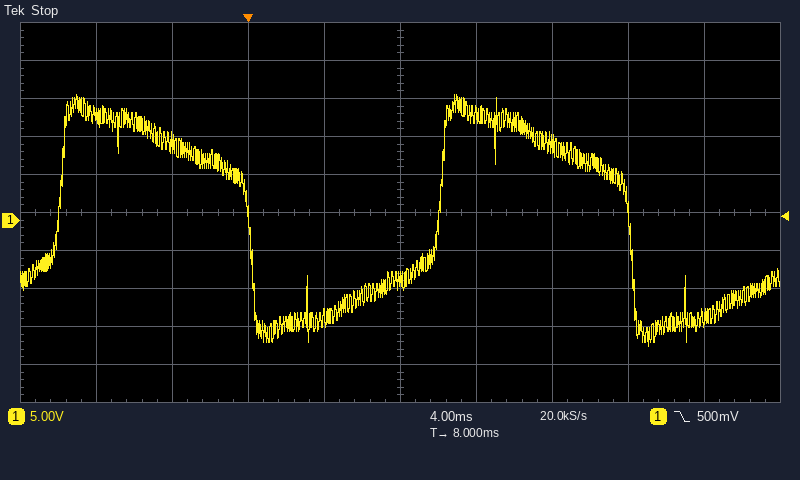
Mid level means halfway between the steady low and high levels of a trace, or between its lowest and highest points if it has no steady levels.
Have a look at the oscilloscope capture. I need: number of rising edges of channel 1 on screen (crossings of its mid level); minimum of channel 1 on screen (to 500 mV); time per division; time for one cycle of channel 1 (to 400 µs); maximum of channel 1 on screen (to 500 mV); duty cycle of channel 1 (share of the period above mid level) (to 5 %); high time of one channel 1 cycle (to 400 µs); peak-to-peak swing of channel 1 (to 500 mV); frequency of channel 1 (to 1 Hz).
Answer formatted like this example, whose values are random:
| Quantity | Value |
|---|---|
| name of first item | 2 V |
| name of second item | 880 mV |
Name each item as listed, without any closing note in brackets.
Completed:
| Quantity | Value |
|---|---|
| number of rising edges of channel 1 on screen | 2 |
| minimum of channel 1 on screen | -16.5 V |
| time per division | 4 ms |
| time for one cycle of channel 1 | 20.0 ms |
| maximum of channel 1 on screen | 16.5 V |
| duty cycle of channel 1 (share of the period above mid level) | 50 % |
| high time of one channel 1 cycle | 10.0 ms |
| peak-to-peak swing of channel 1 | 33.0 V |
| frequency of channel 1 | 50 Hz |
